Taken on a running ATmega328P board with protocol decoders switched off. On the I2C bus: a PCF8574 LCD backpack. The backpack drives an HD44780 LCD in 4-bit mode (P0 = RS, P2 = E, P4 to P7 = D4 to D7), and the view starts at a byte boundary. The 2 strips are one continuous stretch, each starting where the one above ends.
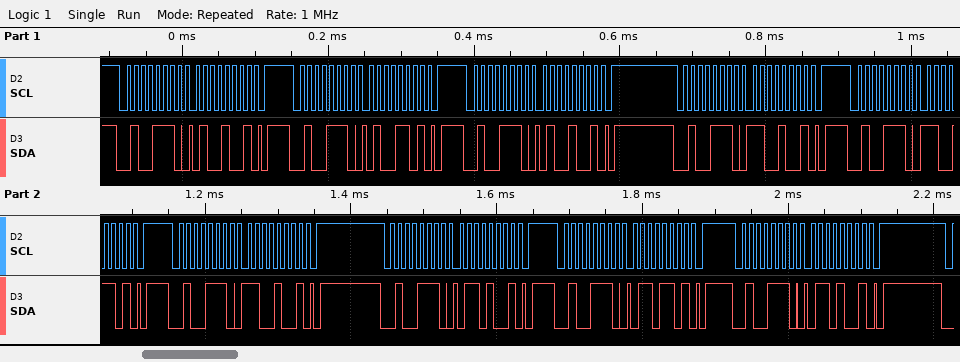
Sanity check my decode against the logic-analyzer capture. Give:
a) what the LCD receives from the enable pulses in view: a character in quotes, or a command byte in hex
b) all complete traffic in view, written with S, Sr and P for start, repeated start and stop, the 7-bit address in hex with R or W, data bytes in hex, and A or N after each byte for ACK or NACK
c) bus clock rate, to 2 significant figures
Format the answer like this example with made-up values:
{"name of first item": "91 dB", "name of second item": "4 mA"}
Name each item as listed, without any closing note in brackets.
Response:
{"what the LCD receives from the enable pulses in view: a character in quotes, or a command byte in hex": "'L'", "all complete traffic in view, written with S, Sr and P for start, repeated start and stop, the 7-bit address in hex with R or W, data bytes in hex, and A or N after each byte for ACK or NACK": "S 27W A 49 A P S 27W A 4D A P S 27W A 49 A P S 27W A C9 A P S 27W A CD A P S 27W A C9 A P S 27W A 69 A P S 27W A 6D A P S 27W A 69 A P", "bus clock rate, to 2 significant figures": "100 kHz"}
